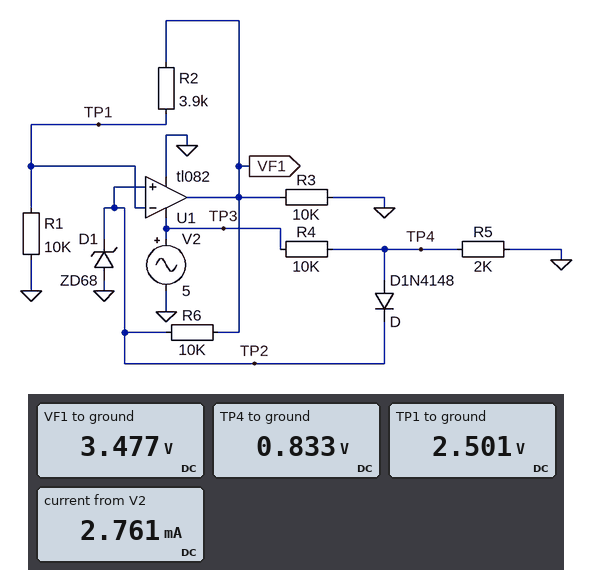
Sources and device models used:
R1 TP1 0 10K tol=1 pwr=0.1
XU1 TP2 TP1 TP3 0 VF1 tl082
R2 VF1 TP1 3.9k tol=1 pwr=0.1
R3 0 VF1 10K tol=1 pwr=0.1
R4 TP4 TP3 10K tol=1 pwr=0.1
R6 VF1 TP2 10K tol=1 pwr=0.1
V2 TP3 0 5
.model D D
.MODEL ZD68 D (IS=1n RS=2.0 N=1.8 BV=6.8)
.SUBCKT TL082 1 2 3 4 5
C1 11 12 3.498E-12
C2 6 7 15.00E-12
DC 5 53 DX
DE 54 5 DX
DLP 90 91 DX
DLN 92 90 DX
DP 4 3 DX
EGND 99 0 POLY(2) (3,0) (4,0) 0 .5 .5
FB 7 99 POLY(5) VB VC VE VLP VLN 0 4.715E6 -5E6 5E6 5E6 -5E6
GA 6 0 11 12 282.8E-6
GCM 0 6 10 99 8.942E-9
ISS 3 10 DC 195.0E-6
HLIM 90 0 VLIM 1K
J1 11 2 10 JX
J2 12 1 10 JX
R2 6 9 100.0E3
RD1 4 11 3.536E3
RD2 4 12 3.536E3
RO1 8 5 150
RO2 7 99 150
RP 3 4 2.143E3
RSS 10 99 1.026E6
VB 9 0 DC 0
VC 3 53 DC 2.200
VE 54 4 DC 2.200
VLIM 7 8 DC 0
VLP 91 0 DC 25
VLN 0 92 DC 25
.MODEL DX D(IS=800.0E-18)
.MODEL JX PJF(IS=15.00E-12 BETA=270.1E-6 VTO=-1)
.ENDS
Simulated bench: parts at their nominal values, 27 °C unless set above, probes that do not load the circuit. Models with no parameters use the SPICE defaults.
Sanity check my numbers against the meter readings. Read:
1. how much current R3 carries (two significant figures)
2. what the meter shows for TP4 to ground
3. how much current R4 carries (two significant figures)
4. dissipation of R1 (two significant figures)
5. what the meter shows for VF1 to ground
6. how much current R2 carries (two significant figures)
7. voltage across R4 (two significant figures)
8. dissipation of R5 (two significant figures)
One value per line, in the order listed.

350 µA
0.833 V
420 µA
630 µW
3.477 V
250 µA
4.2 V
350 µW
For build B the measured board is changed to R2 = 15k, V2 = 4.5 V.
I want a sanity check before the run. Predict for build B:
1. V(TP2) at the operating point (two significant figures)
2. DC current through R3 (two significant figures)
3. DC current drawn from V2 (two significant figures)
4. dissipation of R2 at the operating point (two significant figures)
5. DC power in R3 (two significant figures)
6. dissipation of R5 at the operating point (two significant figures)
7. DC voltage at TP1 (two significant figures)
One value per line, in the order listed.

3.0 V
300 µA
2.5 mA
210 µW
890 µW
280 µW
1.2 V
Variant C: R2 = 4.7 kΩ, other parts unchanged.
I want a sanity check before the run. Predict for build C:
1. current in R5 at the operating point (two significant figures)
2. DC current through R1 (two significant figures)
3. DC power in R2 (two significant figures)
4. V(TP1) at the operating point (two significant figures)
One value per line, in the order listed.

420 µA
240 µA
260 µW
2.4 V
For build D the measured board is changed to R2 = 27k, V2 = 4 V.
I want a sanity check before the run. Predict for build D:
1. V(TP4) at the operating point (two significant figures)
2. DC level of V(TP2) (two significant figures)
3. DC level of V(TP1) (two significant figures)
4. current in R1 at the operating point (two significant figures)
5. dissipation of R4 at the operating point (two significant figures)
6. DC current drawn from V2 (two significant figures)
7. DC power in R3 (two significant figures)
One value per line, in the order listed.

670 mV
2.5 V
690 mV
69 µA
1.1 mW
2.2 mA
610 µW
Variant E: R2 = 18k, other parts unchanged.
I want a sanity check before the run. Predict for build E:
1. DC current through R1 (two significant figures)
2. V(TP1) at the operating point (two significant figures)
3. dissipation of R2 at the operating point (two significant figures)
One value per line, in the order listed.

120 µA
1.2 V
280 µW
